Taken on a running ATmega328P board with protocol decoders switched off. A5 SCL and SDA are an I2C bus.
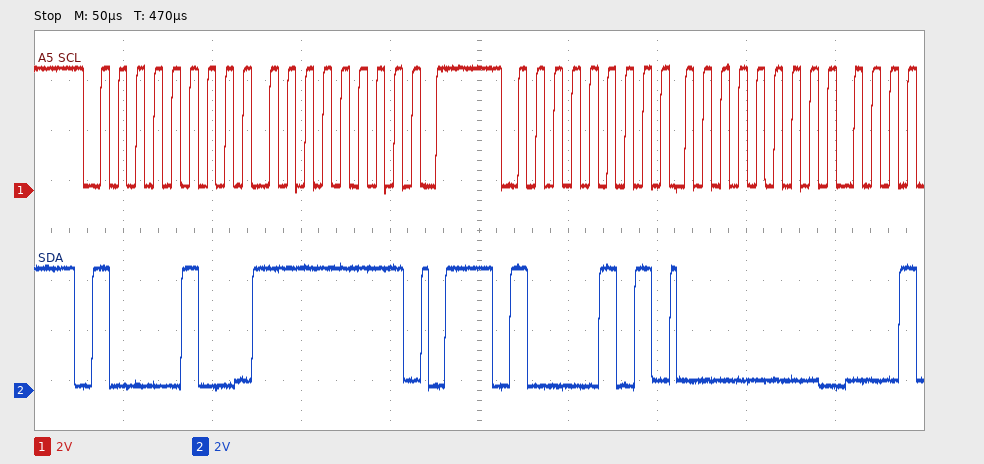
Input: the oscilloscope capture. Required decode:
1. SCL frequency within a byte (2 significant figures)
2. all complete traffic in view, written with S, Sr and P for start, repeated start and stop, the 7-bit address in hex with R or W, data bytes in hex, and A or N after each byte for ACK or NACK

100 kHz
S 42W A FF A P S 42R A 00 A
